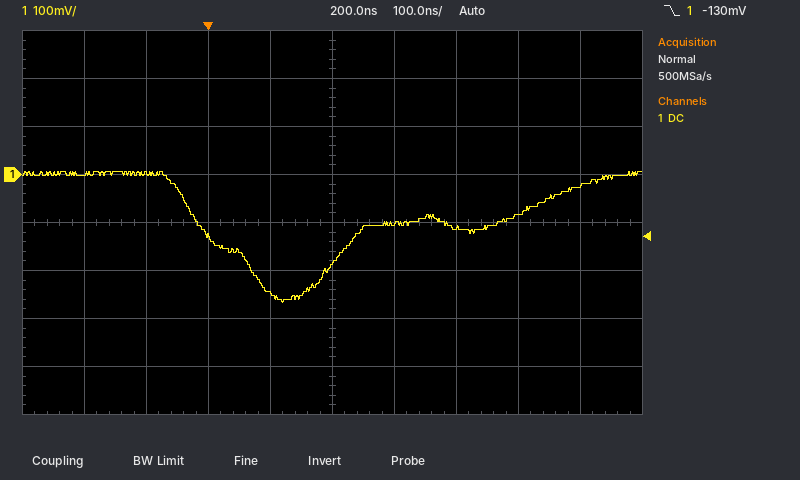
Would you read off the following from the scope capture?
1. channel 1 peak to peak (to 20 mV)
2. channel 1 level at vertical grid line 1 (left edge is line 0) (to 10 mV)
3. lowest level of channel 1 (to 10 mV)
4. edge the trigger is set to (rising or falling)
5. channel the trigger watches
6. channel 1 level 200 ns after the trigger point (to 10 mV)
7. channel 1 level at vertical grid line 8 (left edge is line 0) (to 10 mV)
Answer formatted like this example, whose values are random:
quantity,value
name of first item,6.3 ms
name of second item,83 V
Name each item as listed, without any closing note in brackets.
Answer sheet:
quantity,value
channel 1 peak to peak,280 mV
channel 1 level at vertical grid line 1 (left edge is line 0),0 mV
lowest level of channel 1,-270 mV
edge the trigger is set to,falling
channel the trigger watches,channel 1
channel 1 level 200 ns after the trigger point,-190 mV
channel 1 level at vertical grid line 8 (left edge is line 0),-80 mV
